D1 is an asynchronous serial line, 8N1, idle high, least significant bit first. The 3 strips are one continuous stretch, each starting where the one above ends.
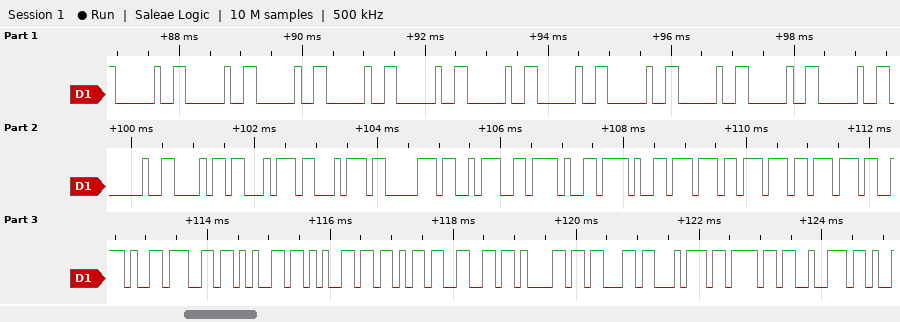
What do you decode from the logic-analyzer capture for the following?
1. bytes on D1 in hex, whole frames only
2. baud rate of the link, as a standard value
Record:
20 20 20 20 20 20 20 20 20 20 20 20 68 74 74 70 3A 2F 2F 77 77 77 2E 67 65 65 6B 66 61 63 74 6F 72
9600 baud
